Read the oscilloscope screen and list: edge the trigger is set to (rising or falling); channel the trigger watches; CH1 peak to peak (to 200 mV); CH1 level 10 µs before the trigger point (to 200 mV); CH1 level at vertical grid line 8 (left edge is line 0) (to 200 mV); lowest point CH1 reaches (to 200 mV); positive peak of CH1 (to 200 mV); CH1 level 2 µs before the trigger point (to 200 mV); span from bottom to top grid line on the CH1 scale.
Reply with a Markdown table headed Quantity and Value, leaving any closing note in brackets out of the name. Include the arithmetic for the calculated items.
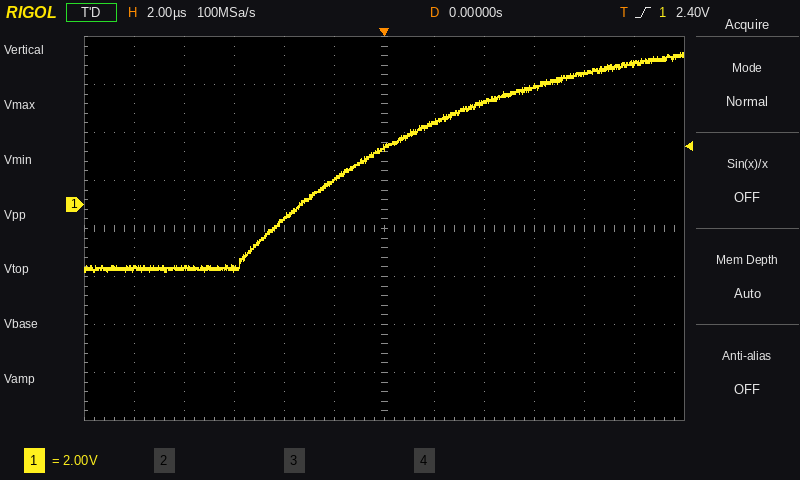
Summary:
| Quantity | Value |
|---|---|
| edge the trigger is set to | rising |
| channel the trigger watches | CH1 |
| CH1 peak to peak | 6.4 V − (-2.8 V) = 9.2 V |
| CH1 level 10 µs before the trigger point | -2.6 V |
| CH1 level at vertical grid line 8 (left edge is line 0) | 4.2 V |
| lowest point CH1 reaches | -2.8 V |
| positive peak of CH1 | 6.4 V |
| CH1 level 2 µs before the trigger point | 1.0 V |
| span from bottom to top grid line on the CH1 scale | 16 V |
